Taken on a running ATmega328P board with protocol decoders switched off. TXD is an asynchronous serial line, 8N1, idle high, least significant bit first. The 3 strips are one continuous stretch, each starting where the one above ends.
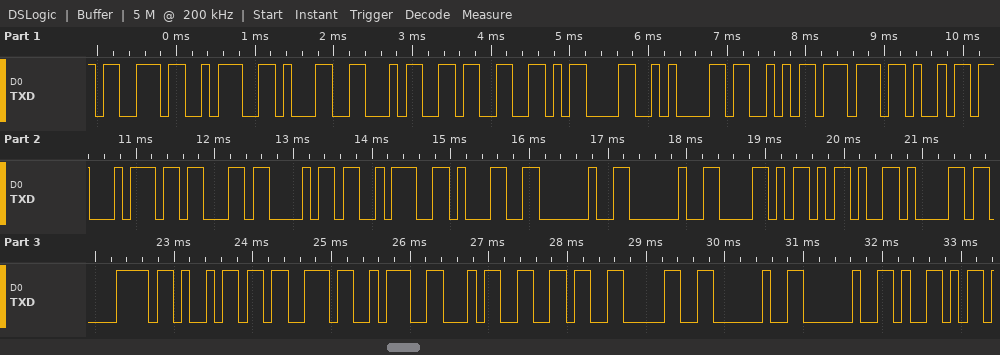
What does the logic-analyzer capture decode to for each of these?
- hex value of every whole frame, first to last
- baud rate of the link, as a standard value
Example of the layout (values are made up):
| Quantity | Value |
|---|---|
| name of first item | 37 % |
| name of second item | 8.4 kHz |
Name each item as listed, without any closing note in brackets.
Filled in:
| Quantity | Value |
|---|---|
| hex value of every whole frame, first to last | 0x73 0x3A 0x31 0x34 0x33 0x0D 0x0A 0x53 0x77 0x69 0x74 0x63 0x68 0x3A 0x31 0x20 0x20 0x58 0x2D 0x61 0x78 0x69 0x73 0x3A 0x34 0x36 0x30 0x20 0x20 0x59 |
| baud rate of the link, as a standard value | 9600 baud |
